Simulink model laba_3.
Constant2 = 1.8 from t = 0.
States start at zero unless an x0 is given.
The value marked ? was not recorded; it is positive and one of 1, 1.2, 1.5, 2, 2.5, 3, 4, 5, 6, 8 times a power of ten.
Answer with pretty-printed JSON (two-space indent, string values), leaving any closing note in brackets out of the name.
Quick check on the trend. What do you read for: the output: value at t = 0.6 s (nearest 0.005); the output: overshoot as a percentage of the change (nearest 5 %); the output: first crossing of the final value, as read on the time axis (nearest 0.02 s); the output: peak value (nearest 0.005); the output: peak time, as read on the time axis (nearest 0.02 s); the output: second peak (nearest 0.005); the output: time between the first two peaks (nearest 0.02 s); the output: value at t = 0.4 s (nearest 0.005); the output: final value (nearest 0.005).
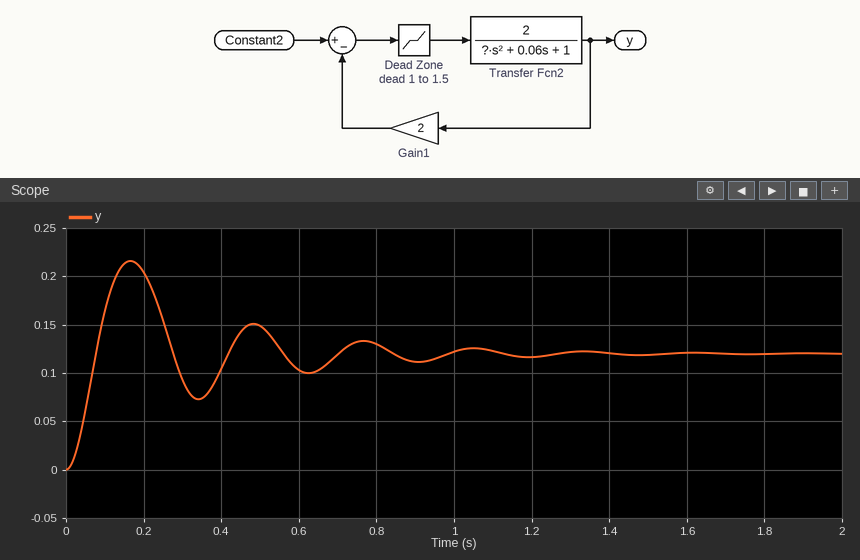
{
  "the output: value at t = 0.6 s": "0.105",
  "the output: overshoot as a percentage of the change": "80 %",
  "the output: first crossing of the final value, as read on the time axis": "0.08 s",
  "the output: peak value": "0.215",
  "the output: peak time, as read on the time axis": "0.16 s",
  "the output: second peak": "0.150",
  "the output: time between the first two peaks": "0.32 s",
  "the output: value at t = 0.4 s": "0.105",
  "the output: final value": "0.120"
}
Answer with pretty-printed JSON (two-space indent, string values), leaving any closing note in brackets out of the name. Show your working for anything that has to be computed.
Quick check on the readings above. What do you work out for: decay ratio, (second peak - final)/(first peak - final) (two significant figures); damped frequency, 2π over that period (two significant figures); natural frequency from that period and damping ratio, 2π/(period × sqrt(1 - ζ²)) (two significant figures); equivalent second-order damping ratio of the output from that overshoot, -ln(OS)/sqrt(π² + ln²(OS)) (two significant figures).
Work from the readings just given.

{
  "decay ratio, (second peak - final)/(first peak - final)": "(0.15 - 0.12) / (0.215 - 0.12) = 0.32",
  "damped frequency, 2π over that period": "2π / 0.32 = 20 rad/s",
  "natural frequency from that period and damping ratio, 2π/(period × sqrt(1 - ζ²))": "2π / (0.32 × sqrt(1 - 0.071²)) = 20 rad/s",
  "equivalent second-order damping ratio of the output from that overshoot, -ln(OS)/sqrt(π² + ln²(OS))": "ln(0.8) = -0.223; 0.223 / sqrt(9.870 + 0.050) = 0.071"
}
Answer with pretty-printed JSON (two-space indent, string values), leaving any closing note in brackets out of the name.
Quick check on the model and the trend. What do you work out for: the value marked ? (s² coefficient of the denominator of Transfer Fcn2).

{
  "the value marked ?": "0.01"
}
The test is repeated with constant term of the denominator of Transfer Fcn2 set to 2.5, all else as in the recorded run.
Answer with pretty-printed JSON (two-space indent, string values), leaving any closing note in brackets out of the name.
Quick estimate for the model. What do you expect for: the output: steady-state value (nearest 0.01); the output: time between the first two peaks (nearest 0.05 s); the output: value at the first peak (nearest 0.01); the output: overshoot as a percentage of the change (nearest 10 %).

{
  "the output: steady-state value": "0.09",
  "the output: time between the first two peaks": "0.25 s",
  "the output: value at the first peak": "0.16",
  "the output: overshoot as a percentage of the change": "70 %"
}
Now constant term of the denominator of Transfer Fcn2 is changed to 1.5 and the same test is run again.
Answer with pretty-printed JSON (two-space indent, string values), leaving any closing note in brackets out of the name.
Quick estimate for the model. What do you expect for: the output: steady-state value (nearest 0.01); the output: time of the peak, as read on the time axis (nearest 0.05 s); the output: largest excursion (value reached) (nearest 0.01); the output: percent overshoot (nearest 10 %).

{
  "the output: steady-state value": "0.11",
  "the output: time of the peak, as read on the time axis": "0.15 s",
  "the output: largest excursion (value reached)": "0.19",
  "the output: percent overshoot": "70 %"
}
